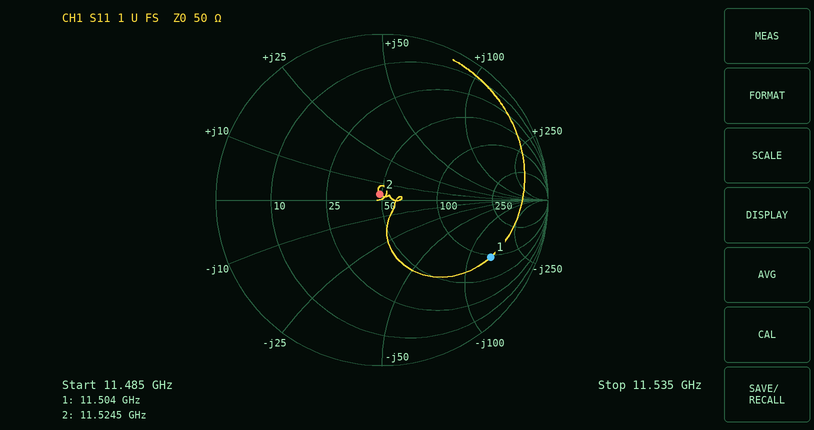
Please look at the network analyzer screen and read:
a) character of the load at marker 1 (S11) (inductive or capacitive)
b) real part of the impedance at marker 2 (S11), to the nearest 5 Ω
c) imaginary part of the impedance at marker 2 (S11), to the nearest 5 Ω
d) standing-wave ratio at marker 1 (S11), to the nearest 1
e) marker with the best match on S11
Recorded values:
capacitive
50 Ω
+5 Ω
7
marker 2
